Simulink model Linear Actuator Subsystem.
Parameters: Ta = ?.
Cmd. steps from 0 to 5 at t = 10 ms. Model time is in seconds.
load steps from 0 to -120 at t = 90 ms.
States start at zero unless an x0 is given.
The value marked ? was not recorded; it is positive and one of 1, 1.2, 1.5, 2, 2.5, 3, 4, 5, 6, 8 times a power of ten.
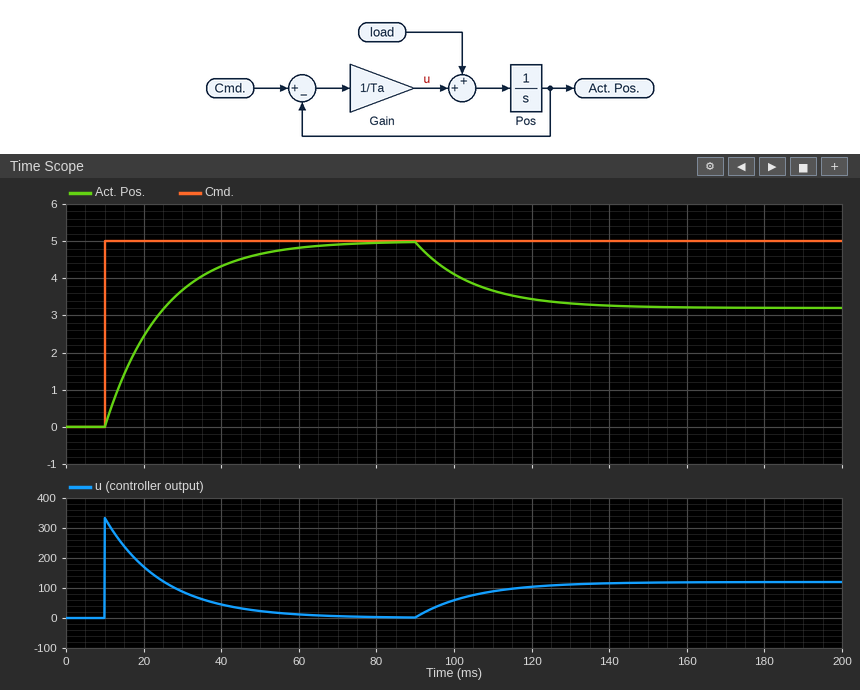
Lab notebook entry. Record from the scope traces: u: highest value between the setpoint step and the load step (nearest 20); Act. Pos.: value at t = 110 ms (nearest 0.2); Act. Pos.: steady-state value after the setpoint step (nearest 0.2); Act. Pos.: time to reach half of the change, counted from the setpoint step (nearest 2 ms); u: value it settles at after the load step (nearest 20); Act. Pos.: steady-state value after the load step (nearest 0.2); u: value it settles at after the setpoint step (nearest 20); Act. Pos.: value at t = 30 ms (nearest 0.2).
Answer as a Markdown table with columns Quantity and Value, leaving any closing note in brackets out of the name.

| Quantity | Value |
|---|---|
| u: highest value between the setpoint step and the load step | 340 |
| Act. Pos.: value at t = 110 ms | 3.6 |
| Act. Pos.: steady-state value after the setpoint step | 5.0 |
| Act. Pos.: time to reach half of the change, counted from the setpoint step | 10 ms |
| u: value it settles at after the load step | 120 |
| Act. Pos.: steady-state value after the load step | 3.2 |
| u: value it settles at after the setpoint step | 0 |
| Act. Pos.: value at t = 30 ms | 3.6 |
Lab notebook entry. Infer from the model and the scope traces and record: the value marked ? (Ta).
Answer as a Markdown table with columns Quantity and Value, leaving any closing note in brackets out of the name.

| Quantity | Value |
|---|---|
| the value marked ? | 0.015 |
